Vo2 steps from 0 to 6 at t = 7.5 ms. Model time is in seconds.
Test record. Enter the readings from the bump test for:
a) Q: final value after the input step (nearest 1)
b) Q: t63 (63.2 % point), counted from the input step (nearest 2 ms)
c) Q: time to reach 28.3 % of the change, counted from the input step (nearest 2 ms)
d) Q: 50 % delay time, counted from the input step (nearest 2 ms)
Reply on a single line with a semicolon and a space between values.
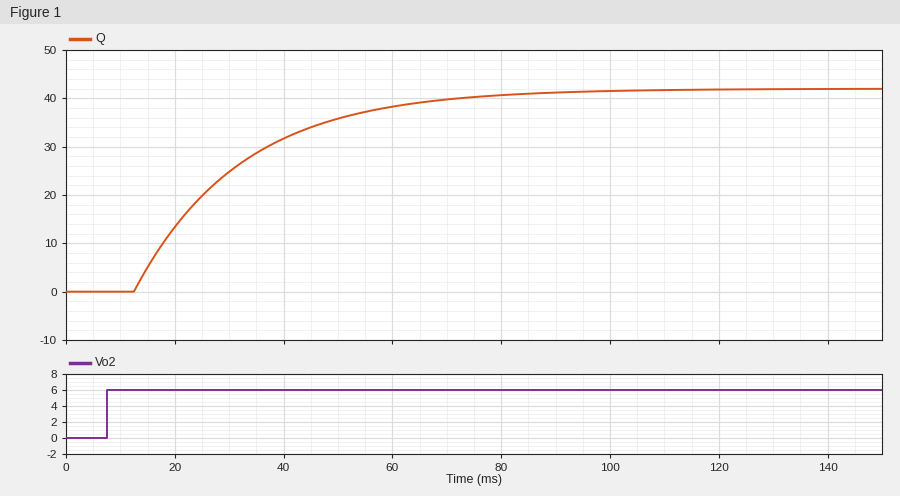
42; 24 ms; 12 ms; 18 ms
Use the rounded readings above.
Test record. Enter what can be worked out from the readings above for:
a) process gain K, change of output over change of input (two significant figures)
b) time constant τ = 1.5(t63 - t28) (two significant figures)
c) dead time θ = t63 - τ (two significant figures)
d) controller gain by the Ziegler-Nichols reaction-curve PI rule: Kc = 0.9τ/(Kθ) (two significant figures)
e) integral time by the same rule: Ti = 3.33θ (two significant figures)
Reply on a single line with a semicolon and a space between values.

7.0; 18 ms; 6.0 ms; 0.39; 20 ms
